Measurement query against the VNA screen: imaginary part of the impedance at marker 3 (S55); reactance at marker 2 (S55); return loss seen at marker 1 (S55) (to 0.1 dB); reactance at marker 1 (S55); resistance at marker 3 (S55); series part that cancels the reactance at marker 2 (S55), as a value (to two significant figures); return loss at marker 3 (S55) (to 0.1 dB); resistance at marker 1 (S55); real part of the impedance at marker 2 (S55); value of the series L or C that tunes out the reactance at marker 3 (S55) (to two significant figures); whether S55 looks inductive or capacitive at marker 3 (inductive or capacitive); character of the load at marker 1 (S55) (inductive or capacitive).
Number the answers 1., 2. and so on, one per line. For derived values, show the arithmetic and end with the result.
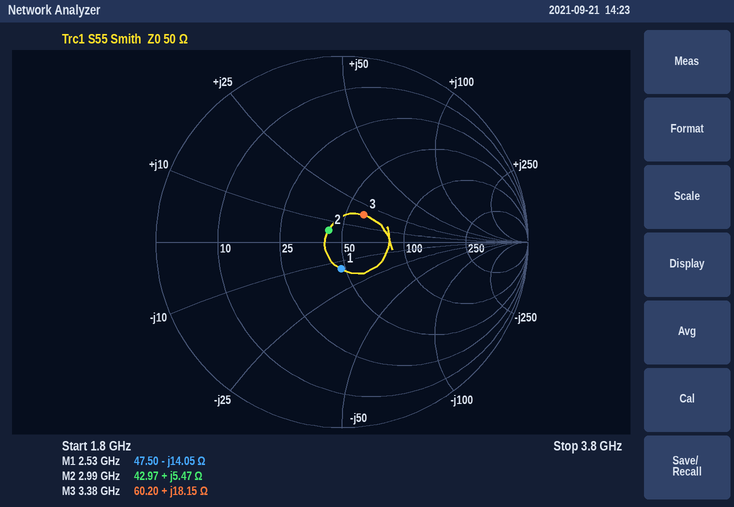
1. +18.15 Ω
2. +5.47 Ω
3. 16.8 dB
4. -14.05 Ω
5. 60.20 Ω
6. C = 1/(2π × 2.99 GHz × 5.47 Ω) ≈ 9.7 pF
7. 14.6 dB
8. 47.50 Ω
9. 42.97 Ω
10. C = 1/(2π × 3.38 GHz × 18.15 Ω) ≈ 2.6 pF
11. inductive
12. capacitive
